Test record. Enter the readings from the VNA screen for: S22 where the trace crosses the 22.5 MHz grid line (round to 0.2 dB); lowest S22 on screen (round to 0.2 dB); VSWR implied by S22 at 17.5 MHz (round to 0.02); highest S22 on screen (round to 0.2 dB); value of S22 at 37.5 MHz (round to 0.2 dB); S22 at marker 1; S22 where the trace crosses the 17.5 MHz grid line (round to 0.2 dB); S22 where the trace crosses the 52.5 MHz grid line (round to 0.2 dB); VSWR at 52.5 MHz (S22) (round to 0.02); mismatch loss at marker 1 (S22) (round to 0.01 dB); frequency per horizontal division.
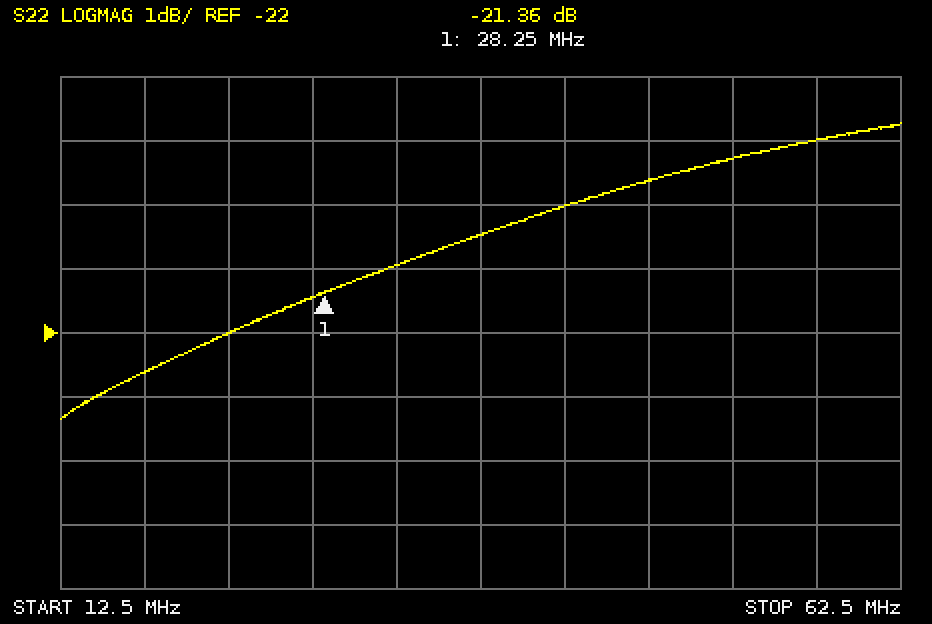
-22.0 dB
-23.4 dB
1.16
-18.8 dB
-20.4 dB
-21.36 dB
-22.6 dB
-19.2 dB
1.24
0.03 dB
5 MHz
